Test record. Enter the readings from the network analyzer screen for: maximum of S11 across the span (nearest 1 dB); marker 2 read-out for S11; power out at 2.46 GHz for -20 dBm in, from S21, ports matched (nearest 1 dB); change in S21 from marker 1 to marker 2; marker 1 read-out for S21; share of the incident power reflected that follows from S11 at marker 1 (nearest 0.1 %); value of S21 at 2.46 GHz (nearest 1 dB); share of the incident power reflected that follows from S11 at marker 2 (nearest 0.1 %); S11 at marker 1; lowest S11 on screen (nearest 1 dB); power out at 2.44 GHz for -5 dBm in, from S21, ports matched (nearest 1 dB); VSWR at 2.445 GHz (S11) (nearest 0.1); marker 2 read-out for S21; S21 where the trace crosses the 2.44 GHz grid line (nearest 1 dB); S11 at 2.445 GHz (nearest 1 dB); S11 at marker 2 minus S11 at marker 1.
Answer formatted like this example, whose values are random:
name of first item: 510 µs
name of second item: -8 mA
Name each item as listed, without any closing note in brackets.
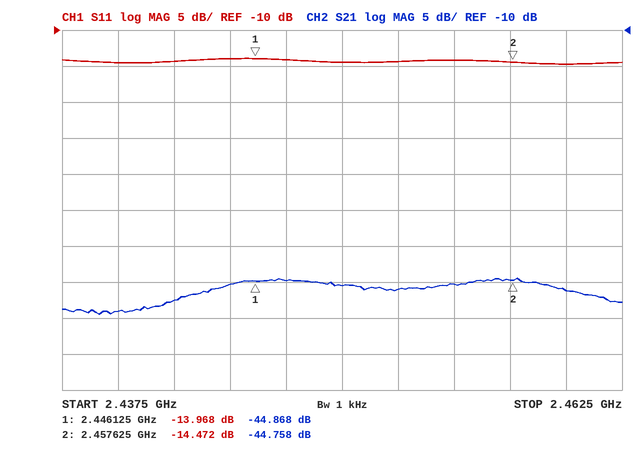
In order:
maximum of S11 across the span: -14 dB
marker 2 read-out for S11: -14.472 dB
power out at 2.46 GHz for -20 dBm in, from S21, ports matched: -66 dBm
change in S21 from marker 1 to marker 2: 0.110 dB
marker 1 read-out for S21: -44.868 dB
share of the incident power reflected that follows from S11 at marker 1: 4.0 %
value of S21 at 2.46 GHz: -46 dB
share of the incident power reflected that follows from S11 at marker 2: 3.6 %
S11 at marker 1: -13.968 dB
lowest S11 on screen: -15 dB
power out at 2.44 GHz for -5 dBm in, from S21, ports matched: -54 dBm
VSWR at 2.445 GHz (S11): 1.5
marker 2 read-out for S21: -44.758 dB
S21 where the trace crosses the 2.44 GHz grid line: -49 dB
S11 at 2.445 GHz: -14 dB
S11 at marker 2 minus S11 at marker 1: -0.504 dB
